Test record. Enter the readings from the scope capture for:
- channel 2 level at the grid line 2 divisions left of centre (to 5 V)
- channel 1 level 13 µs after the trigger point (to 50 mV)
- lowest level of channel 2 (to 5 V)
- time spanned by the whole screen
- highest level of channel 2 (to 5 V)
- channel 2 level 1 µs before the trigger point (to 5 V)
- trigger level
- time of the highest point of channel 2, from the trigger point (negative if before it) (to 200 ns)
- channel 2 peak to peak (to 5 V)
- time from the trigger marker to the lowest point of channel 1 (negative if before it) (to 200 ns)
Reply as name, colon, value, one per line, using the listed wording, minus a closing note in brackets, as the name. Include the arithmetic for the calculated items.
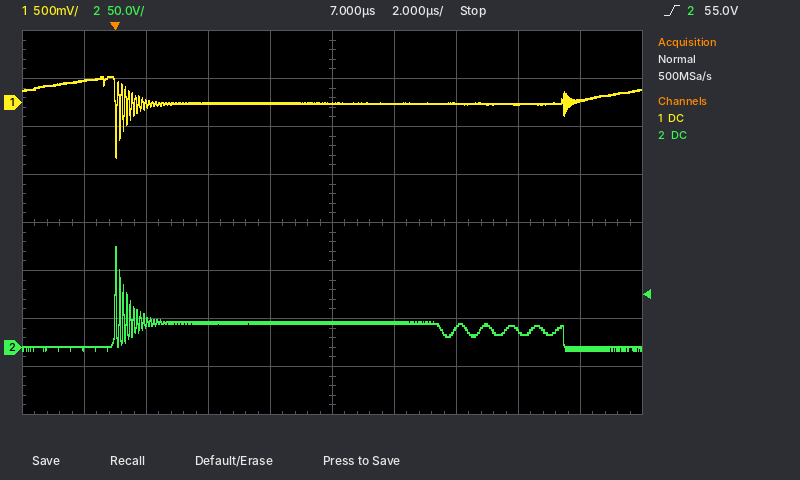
channel 2 level at the grid line 2 divisions left of centre: 25 V
channel 1 level 13 µs after the trigger point: 0 mV
lowest level of channel 2: -5 V
time spanned by the whole screen: 20 µs
highest level of channel 2: 105 V
channel 2 level 1 µs before the trigger point: 0 V
trigger level: 55.0 V
time of the highest point of channel 2, from the trigger point (negative if before it): 0.0 µs
channel 2 peak to peak: 105 V − (-5 V) = 110 V
time from the trigger marker to the lowest point of channel 1 (negative if before it): 0.0 µs
